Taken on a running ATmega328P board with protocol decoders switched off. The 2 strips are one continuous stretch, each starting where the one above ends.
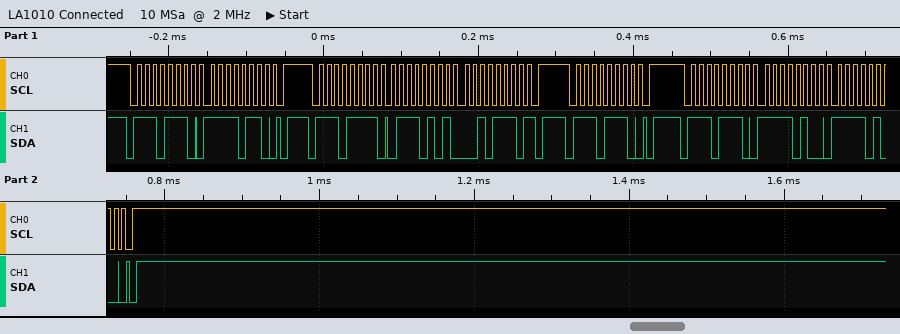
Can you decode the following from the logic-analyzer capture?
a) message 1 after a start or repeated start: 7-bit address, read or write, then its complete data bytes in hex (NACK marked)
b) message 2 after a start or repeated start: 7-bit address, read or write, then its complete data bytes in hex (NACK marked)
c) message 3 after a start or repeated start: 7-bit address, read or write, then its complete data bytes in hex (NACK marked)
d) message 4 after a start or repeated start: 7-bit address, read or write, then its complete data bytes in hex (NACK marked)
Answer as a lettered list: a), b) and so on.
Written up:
a) 0x77 write: F6
b) 0x77 read: 75 2E NACK
c) 0x77 write
d) 0x77 write: F4 F4
